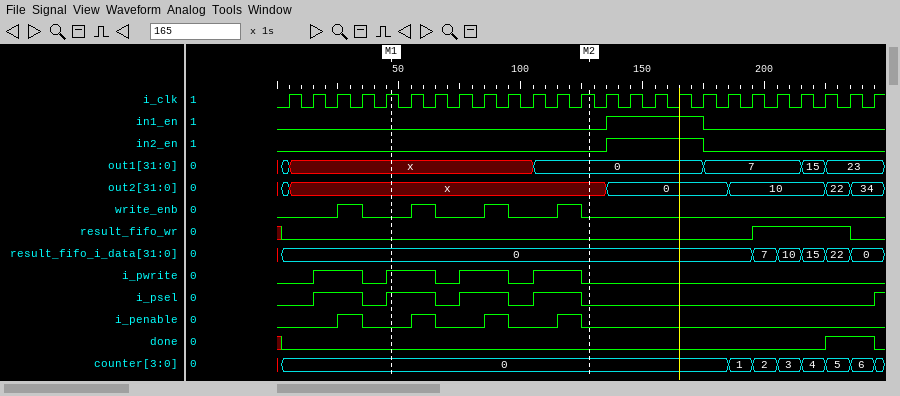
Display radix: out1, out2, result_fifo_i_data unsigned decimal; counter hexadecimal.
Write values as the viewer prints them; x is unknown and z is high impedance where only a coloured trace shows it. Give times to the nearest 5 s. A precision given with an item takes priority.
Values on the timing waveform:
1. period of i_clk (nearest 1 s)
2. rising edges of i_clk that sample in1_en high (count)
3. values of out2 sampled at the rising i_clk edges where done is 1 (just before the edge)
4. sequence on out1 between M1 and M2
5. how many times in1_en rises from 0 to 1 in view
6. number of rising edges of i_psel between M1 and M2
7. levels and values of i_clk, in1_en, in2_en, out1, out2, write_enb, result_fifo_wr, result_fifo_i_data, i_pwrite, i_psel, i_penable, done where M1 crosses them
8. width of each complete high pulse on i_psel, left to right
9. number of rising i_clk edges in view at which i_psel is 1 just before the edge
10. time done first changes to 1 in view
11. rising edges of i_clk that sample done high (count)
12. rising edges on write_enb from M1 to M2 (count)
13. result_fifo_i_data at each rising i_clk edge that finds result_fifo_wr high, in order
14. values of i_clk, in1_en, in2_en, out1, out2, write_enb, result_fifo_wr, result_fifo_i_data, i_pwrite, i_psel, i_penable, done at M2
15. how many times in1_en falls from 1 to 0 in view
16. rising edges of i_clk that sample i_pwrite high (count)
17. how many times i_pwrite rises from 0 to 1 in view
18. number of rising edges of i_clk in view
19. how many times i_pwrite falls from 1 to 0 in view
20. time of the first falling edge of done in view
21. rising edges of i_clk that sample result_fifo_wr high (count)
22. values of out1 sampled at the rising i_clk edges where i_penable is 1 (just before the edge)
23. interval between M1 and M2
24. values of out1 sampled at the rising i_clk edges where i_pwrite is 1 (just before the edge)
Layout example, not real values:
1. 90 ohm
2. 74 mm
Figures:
1. 10 s
2. 4
3. 22, 34
4. x, 0
5. 1
6. 2
7. i_clk=1, in1_en=0, in2_en=0, out1=x, out2=x, write_enb=0, result_fifo_wr=0, result_fifo_i_data=0, i_pwrite=1, i_psel=1, i_penable=0, done=0
8. 20 s, 20 s, 20 s, 20 s
9. 8
10. 225 s
11. 2
12. 3
13. 7, 10, 15, 22
14. i_clk=1, in1_en=0, in2_en=0, out1=0, out2=x, write_enb=0, result_fifo_wr=0, result_fifo_i_data=0, i_pwrite=0, i_psel=0, i_penable=0, done=0
15. 1
16. 8
17. 4
18. 25
19. 4
20. 245 s
21. 4
22. x, x, x, 0
23. 80 s
24. x, x, x, x, x, x, 0, 0
